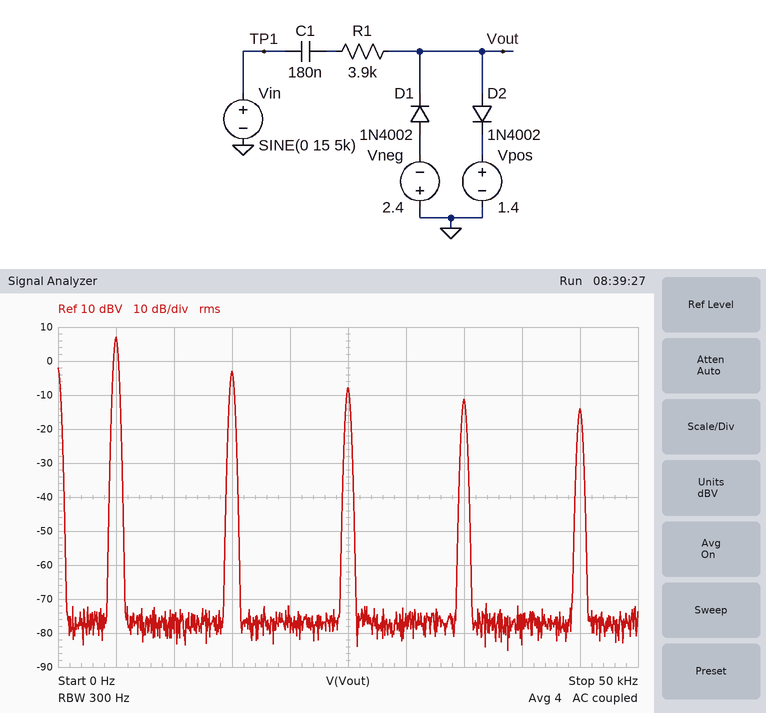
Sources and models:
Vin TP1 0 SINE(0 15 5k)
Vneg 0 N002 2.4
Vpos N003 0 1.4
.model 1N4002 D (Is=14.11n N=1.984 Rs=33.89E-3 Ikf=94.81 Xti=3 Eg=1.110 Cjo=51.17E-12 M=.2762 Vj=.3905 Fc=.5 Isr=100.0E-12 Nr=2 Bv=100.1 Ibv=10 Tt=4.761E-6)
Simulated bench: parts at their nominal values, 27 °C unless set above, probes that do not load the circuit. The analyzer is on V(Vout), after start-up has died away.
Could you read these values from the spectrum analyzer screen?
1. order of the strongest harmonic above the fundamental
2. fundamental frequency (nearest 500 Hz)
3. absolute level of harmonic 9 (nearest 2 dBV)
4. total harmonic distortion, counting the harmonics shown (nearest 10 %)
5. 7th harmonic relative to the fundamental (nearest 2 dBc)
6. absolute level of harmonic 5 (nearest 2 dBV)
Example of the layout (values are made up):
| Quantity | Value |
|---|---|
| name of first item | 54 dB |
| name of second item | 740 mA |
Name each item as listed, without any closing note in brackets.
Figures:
| Quantity | Value |
|---|---|
| order of the strongest harmonic above the fundamental | 3 |
| fundamental frequency | 5.0 kHz |
| absolute level of harmonic 9 | -14 dBV |
| total harmonic distortion, counting the harmonics shown | 40 % |
| 7th harmonic relative to the fundamental | -18 dBc |
| absolute level of harmonic 5 | -8 dBV |
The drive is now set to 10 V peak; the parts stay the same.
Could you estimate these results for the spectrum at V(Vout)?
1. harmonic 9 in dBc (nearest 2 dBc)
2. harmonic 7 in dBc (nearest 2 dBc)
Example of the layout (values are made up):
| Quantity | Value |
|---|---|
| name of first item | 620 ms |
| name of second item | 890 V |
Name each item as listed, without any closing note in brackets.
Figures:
| Quantity | Value |
|---|---|
| harmonic 9 in dBc | -24 dBc |
| harmonic 7 in dBc | -20 dBc |
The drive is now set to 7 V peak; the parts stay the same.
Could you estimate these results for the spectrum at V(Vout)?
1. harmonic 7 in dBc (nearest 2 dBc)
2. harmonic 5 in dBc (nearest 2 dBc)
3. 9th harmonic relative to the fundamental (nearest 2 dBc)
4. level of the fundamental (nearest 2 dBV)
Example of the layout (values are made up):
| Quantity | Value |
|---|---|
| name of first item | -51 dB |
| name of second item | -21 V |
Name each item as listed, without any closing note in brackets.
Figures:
| Quantity | Value |
|---|---|
| harmonic 7 in dBc | -26 dBc |
| harmonic 5 in dBc | -18 dBc |
| 9th harmonic relative to the fundamental | -36 dBc |
| level of the fundamental | 6 dBV |
